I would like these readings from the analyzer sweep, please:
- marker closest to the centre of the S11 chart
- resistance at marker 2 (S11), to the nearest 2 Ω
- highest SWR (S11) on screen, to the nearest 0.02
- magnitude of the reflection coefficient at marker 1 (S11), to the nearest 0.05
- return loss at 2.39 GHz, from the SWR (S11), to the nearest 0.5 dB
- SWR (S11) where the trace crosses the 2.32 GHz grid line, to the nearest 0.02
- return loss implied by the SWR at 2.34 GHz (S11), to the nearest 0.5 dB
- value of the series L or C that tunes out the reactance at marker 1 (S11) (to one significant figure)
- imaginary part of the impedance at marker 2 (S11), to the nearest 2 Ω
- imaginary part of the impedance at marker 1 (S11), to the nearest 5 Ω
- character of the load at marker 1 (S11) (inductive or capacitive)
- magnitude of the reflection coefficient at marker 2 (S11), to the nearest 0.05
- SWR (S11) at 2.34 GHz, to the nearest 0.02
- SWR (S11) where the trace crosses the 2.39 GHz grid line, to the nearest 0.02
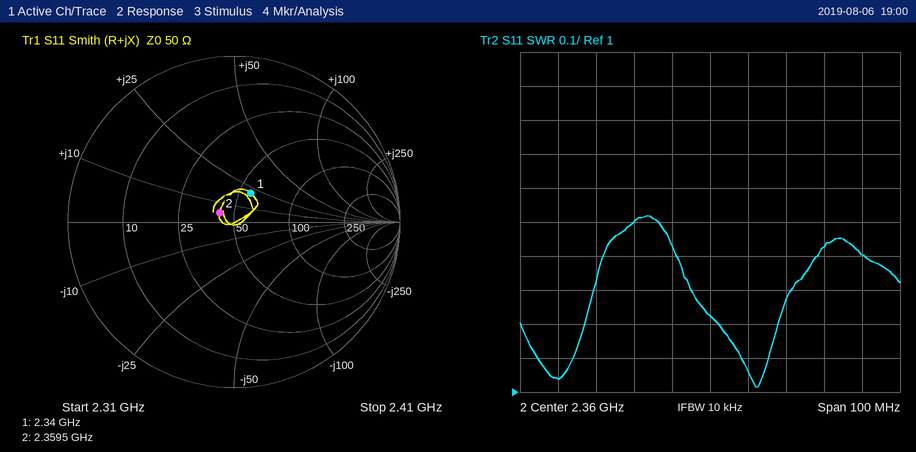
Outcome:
marker 2
42 Ω
1.52
0.20
15.0 dB
1.04
14.0 dB
3 pF
+4 Ω
+20 Ω
inductive
0.10
1.50
1.42
